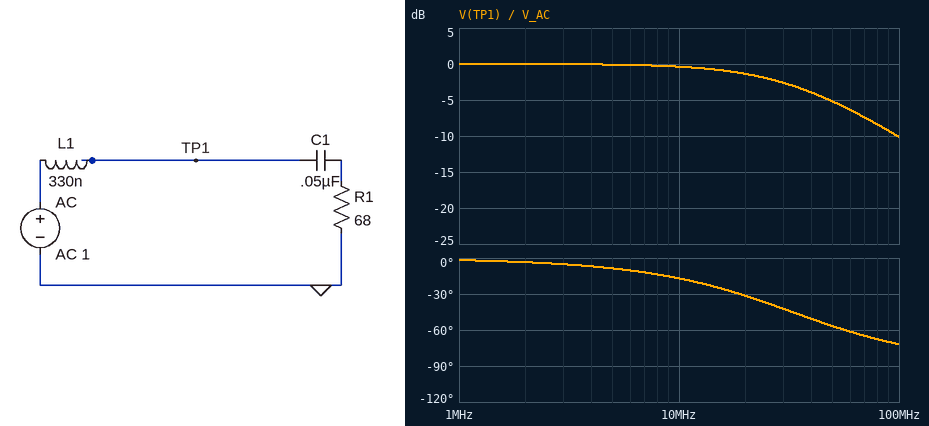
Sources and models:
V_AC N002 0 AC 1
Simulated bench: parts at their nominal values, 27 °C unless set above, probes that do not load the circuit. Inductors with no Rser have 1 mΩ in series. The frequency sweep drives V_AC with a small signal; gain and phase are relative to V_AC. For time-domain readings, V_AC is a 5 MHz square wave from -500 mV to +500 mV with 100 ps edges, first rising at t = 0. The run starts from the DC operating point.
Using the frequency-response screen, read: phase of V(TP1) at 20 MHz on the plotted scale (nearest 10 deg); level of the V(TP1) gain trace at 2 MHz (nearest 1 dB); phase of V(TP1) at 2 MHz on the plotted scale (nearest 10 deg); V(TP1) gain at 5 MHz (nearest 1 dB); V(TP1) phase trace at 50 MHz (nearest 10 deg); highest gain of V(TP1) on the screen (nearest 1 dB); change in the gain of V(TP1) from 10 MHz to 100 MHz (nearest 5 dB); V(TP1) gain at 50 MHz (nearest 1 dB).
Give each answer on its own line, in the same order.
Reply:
-30 deg
0 dB
0 deg
0 dB
-60 deg
0 dB
-10 dB
-5 dB
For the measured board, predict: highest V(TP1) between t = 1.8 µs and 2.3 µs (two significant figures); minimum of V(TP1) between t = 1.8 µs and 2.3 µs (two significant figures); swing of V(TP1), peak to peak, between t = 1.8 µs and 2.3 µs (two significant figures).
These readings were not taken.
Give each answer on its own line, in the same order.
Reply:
500 mV
-500 mV
1.0 V
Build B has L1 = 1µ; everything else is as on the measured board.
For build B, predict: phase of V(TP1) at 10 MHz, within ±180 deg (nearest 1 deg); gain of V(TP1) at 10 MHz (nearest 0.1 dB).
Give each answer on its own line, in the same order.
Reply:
-43 deg
-2.7 dB
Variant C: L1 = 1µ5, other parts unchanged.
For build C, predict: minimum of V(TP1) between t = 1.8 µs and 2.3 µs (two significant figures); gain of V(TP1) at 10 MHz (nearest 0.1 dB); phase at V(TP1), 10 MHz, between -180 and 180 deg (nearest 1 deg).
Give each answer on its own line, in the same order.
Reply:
-490 mV
-4.6 dB
-54 deg
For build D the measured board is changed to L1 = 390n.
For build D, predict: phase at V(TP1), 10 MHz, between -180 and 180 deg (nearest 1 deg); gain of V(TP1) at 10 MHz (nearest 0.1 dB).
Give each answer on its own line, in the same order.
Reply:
-20 deg
-0.5 dB
